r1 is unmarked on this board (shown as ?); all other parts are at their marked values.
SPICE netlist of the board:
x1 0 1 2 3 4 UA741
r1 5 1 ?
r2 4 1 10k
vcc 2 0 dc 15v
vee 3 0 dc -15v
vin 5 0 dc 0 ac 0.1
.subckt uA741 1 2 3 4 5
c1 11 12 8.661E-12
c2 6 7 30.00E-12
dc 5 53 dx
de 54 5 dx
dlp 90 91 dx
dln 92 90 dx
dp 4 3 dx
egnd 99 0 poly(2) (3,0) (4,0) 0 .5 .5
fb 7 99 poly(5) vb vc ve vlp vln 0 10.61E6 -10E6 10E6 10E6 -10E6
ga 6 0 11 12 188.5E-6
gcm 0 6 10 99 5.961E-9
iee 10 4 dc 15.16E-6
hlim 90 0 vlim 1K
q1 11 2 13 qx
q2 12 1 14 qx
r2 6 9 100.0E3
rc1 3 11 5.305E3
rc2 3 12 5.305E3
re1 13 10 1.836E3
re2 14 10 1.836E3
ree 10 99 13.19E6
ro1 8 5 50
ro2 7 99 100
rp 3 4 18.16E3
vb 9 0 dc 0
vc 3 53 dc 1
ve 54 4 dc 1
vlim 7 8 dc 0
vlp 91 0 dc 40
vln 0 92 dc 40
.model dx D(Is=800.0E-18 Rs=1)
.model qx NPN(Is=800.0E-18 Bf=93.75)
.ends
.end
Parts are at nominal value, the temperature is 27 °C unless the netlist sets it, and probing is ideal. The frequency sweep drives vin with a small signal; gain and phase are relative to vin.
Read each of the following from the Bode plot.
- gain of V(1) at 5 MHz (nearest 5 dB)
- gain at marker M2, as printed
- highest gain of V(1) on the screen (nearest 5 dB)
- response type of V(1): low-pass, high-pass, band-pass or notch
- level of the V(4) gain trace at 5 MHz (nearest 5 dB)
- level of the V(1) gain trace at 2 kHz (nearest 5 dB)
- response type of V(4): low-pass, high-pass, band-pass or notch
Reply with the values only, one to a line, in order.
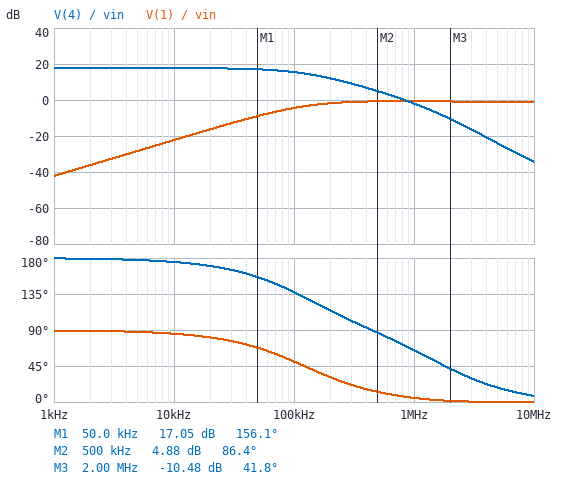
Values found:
0 dB
4.88 dB
0 dB
high-pass
-25 dB
-35 dB
low-pass
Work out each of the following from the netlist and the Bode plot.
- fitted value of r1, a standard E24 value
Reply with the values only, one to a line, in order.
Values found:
1.3 kΩ
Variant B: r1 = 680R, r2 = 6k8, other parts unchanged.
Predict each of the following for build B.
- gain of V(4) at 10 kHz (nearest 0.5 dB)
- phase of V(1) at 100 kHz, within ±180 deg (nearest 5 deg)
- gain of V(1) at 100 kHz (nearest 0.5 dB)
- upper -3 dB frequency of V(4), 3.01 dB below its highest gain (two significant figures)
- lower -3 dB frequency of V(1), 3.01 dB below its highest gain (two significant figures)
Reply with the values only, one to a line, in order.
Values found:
20.0 dB
45 deg
-3.0 dB
95 kHz
92 kHz
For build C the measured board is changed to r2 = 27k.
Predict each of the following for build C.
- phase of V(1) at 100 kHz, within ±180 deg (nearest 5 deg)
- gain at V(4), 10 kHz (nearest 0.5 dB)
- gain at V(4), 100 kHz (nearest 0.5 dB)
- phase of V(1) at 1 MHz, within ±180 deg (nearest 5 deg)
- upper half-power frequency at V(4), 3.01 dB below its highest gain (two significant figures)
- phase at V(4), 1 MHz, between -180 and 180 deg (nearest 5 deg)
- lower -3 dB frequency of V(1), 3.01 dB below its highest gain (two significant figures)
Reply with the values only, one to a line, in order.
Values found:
25 deg
26.0 dB
19.0 dB
0 deg
47 kHz
60 deg
46 kHz
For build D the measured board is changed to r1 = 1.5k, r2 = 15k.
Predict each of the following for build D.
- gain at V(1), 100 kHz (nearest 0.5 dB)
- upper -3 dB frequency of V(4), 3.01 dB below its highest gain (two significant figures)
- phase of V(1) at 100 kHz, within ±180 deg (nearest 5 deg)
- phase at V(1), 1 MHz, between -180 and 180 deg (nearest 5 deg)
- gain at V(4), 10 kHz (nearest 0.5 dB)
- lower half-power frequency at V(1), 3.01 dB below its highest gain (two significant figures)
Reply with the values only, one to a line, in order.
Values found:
-3.0 dB
95 kHz
45 deg
5 deg
20.0 dB
92 kHz
